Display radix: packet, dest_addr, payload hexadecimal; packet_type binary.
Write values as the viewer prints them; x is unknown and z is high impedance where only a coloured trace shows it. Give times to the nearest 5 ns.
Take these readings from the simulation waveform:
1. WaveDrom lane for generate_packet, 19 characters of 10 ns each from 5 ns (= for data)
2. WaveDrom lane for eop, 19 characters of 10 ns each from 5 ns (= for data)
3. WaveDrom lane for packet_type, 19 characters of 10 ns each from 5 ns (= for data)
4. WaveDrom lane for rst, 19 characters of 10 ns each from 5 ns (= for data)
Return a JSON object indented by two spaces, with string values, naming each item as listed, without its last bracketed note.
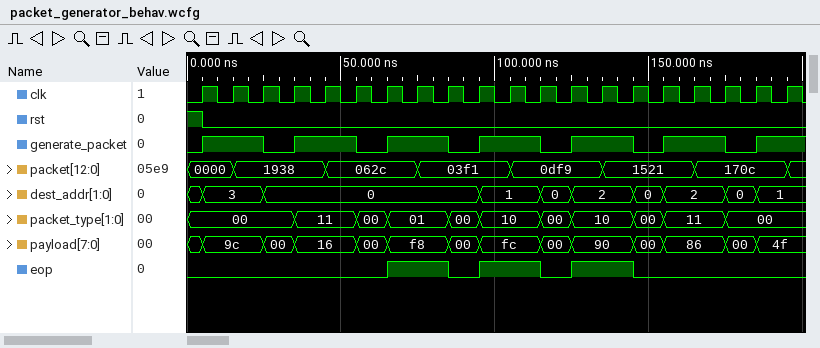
{
  "WaveDrom lane for generate_packet, 19 characters of 10 ns each from 5 ns": "{name: 'generate_packet', wave: '1.01.01.01.01.01.01'}",
  "WaveDrom lane for eop, 19 characters of 10 ns each from 5 ns": "{name: 'eop', wave: '0.....1.01.01.0....'}",
  "WaveDrom lane for packet_type, 19 characters of 10 ns each from 5 ns": "{name: 'packet_type', wave: '=..=.==.==.==.==.=.', data: '00 11 00 01 00 10 00 10 00 11 00'}",
  "WaveDrom lane for rst, 19 characters of 10 ns each from 5 ns": "{name: 'rst', wave: '0..................'}"
}
